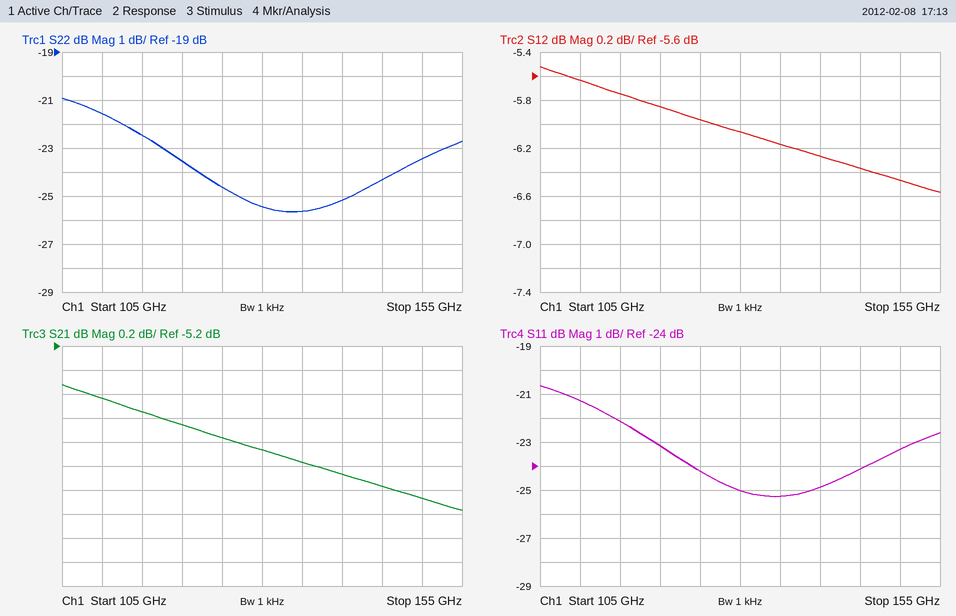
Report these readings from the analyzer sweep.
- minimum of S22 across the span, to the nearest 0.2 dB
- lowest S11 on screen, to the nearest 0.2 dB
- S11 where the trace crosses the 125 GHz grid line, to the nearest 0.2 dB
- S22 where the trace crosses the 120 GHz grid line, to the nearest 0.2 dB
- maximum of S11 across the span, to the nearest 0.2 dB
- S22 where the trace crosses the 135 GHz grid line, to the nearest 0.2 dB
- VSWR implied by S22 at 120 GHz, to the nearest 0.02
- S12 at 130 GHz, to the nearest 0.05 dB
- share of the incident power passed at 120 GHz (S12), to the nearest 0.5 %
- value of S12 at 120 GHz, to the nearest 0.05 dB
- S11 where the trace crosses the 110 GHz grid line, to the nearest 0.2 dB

-25.6 dB
-25.2 dB
-24.2 dB
-23.6 dB
-20.6 dB
-25.6 dB
1.14
-6.05 dB
26.0 %
-5.85 dB
-21.2 dB
